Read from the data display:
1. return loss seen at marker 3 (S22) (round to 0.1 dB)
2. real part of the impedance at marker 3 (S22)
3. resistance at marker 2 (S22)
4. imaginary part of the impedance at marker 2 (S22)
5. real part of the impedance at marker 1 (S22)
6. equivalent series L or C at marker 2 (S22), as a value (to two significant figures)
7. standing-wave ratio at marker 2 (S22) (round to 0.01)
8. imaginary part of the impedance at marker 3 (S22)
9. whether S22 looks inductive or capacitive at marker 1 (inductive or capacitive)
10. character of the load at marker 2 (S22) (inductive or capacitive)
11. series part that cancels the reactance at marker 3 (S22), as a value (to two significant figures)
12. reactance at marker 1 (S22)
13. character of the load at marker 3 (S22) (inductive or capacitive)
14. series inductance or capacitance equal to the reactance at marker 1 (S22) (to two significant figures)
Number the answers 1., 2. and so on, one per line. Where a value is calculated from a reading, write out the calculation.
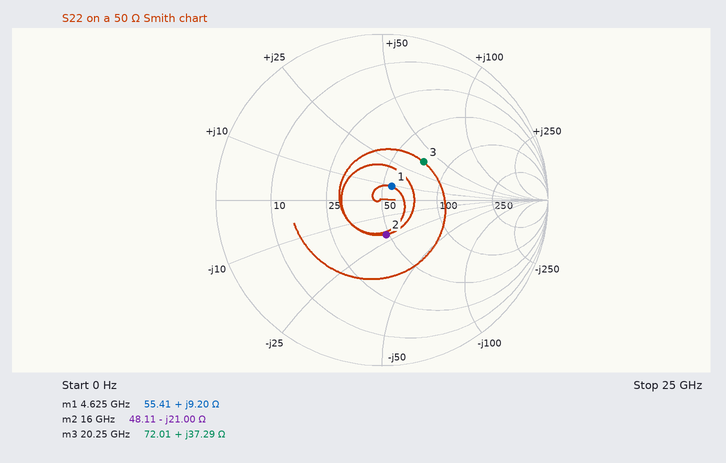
1. 9.4 dB
2. 72.01 Ω
3. 48.11 Ω
4. -21.00 Ω
5. 55.41 Ω
6. C = 1/(2π × 16 GHz × 21 Ω) ≈ 474 fF, so 470 fF to two significant figures
7. 1.53
8. +37.29 Ω
9. inductive
10. capacitive
11. C = 1/(2π × 20.25 GHz × 37.29 Ω) ≈ 211 fF, so 210 fF to two significant figures
12. +9.20 Ω
13. inductive
14. L = 9.2 Ω/(2π × 4.625 GHz) ≈ 317 pH, so 320 pH to two significant figures
